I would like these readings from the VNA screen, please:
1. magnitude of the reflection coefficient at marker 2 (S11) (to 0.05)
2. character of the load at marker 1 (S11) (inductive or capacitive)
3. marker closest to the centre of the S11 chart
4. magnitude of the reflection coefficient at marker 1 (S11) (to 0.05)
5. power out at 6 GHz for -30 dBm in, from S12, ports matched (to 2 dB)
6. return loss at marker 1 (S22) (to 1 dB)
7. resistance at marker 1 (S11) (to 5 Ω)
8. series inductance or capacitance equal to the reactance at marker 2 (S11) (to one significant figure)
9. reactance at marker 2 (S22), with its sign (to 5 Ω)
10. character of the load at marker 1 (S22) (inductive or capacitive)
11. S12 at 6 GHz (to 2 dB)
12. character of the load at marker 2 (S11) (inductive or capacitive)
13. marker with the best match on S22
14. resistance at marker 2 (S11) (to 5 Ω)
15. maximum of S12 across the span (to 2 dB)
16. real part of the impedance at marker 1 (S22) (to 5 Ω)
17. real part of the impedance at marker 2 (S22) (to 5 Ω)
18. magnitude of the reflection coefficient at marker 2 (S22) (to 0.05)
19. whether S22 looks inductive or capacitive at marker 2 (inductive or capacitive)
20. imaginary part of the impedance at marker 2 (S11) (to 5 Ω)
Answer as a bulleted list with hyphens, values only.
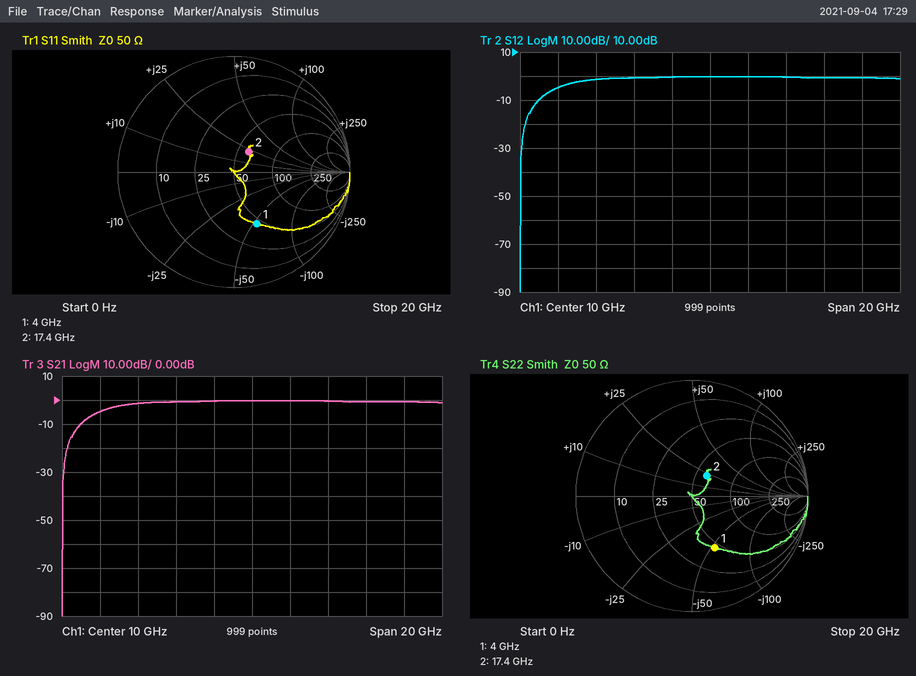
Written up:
- 0.20
- capacitive
- marker 2
- 0.50
- -30 dBm
- 6 dB
- 45 Ω
- 200 pH
- +20 Ω
- capacitive
- 0 dB
- inductive
- marker 2
- 60 Ω
- 0 dB
- 45 Ω
- 60 Ω
- 0.20
- inductive
- +20 Ω
